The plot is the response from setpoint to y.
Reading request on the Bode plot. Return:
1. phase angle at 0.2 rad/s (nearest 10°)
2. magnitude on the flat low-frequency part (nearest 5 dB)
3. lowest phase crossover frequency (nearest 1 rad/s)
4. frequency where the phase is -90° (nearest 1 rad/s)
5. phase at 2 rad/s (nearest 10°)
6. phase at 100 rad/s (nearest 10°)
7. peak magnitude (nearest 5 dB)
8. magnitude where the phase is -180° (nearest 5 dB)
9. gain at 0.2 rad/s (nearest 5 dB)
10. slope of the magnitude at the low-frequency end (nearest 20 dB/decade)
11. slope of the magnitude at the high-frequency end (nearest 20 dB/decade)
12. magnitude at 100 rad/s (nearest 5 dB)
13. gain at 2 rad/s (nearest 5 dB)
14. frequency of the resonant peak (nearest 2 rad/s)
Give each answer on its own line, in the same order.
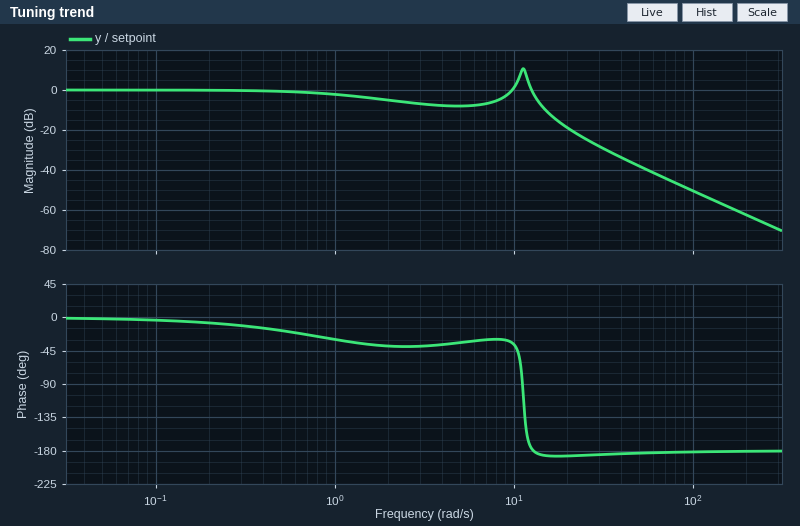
-10°
0 dB
13 rad/s
11 rad/s
-40°
-180°
10 dB
0 dB
0 dB
0 dB/decade
-40 dB/decade
-50 dB
-5 dB
12 rad/s
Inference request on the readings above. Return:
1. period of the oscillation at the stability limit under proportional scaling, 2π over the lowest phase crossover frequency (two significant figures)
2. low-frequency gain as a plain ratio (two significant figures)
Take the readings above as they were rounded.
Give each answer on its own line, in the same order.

0.48 s
1.0
